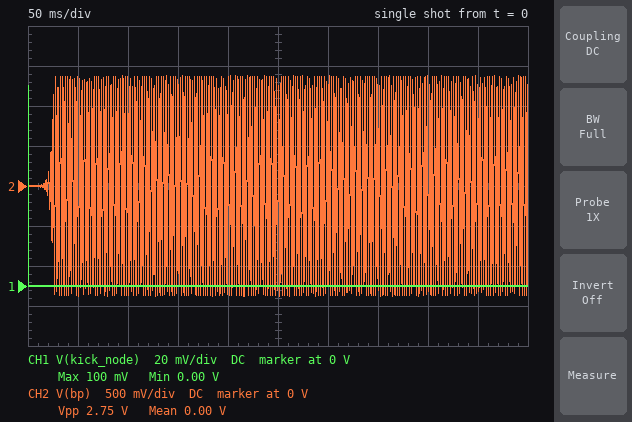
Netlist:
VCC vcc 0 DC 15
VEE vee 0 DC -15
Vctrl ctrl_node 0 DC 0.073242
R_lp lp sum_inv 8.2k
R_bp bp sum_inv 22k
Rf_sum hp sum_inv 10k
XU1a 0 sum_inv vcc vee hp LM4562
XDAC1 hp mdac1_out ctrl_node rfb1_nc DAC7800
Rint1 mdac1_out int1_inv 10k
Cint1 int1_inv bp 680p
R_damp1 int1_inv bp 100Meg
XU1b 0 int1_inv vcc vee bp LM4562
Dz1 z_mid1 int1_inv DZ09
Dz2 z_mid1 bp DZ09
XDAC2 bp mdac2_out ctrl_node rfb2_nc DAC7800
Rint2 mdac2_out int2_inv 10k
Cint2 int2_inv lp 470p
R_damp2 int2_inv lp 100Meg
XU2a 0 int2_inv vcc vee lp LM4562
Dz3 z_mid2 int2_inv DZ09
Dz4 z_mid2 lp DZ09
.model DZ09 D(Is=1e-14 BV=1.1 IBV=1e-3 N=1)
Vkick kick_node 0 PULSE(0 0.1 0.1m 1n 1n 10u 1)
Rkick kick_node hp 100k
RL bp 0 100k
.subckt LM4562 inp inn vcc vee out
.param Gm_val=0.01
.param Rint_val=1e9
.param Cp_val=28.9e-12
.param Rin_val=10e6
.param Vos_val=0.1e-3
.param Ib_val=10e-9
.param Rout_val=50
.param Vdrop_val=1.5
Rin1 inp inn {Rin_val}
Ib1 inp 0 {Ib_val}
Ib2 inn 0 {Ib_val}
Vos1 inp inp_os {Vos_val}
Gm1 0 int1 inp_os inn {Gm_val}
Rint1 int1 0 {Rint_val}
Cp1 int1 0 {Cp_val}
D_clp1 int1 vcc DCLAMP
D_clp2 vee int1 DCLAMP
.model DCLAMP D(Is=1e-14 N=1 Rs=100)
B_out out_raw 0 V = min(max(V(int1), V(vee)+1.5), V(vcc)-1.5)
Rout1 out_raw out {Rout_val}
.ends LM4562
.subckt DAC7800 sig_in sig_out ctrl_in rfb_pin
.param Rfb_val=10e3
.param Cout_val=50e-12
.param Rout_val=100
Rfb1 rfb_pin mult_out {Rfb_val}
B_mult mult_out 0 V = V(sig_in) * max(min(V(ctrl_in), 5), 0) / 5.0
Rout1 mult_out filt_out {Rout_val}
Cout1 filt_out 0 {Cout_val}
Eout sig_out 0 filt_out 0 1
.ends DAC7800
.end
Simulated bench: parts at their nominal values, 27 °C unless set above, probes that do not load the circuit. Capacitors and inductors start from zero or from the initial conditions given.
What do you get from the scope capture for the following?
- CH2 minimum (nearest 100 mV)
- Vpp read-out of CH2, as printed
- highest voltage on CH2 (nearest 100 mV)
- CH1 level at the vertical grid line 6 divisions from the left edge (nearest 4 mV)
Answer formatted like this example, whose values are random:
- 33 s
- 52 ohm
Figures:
- -1.4 V
- 2.75 V
- 1.4 V
- 0 V
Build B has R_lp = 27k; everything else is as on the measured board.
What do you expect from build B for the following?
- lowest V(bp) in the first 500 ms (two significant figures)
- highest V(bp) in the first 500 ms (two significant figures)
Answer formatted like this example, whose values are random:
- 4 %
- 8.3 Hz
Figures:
- -1.1 V
- 1.1 V
